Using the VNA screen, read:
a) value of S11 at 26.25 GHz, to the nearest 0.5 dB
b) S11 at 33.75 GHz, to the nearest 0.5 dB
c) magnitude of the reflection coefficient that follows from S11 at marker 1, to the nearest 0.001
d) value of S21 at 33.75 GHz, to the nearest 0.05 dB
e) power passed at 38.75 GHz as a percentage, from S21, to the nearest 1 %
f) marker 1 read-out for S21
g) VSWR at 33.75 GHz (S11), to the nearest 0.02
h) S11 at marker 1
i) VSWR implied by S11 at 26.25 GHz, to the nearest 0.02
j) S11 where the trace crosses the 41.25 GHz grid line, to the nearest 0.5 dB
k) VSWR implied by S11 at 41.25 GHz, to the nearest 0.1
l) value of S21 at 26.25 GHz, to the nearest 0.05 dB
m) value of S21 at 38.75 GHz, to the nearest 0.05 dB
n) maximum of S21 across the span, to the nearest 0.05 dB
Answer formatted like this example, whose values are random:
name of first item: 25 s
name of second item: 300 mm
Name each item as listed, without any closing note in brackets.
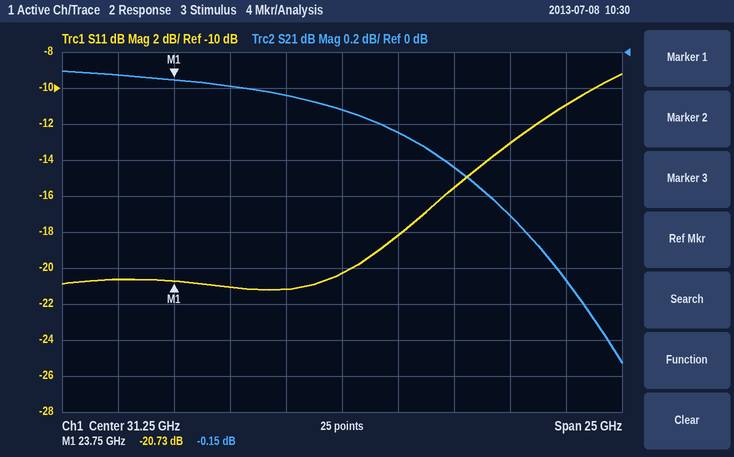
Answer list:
value of S11 at 26.25 GHz, to the nearest 0.5 dB: -21.0 dB
S11 at 33.75 GHz, to the nearest 0.5 dB: -18.0 dB
magnitude of the reflection coefficient that follows from S11 at marker 1, to the nearest 0.001: 0.092
value of S21 at 33.75 GHz, to the nearest 0.05 dB: -0.45 dB
power passed at 38.75 GHz as a percentage, from S21, to the nearest 1 %: 81 %
marker 1 read-out for S21: -0.15 dB
VSWR at 33.75 GHz (S11), to the nearest 0.02: 1.28
S11 at marker 1: -20.73 dB
VSWR implied by S11 at 26.25 GHz, to the nearest 0.02: 1.20
S11 where the trace crosses the 41.25 GHz grid line, to the nearest 0.5 dB: -11.0 dB
VSWR implied by S11 at 41.25 GHz, to the nearest 0.1: 1.8
value of S21 at 26.25 GHz, to the nearest 0.05 dB: -0.20 dB
value of S21 at 38.75 GHz, to the nearest 0.05 dB: -0.90 dB
maximum of S21 across the span, to the nearest 0.05 dB: -0.10 dB
